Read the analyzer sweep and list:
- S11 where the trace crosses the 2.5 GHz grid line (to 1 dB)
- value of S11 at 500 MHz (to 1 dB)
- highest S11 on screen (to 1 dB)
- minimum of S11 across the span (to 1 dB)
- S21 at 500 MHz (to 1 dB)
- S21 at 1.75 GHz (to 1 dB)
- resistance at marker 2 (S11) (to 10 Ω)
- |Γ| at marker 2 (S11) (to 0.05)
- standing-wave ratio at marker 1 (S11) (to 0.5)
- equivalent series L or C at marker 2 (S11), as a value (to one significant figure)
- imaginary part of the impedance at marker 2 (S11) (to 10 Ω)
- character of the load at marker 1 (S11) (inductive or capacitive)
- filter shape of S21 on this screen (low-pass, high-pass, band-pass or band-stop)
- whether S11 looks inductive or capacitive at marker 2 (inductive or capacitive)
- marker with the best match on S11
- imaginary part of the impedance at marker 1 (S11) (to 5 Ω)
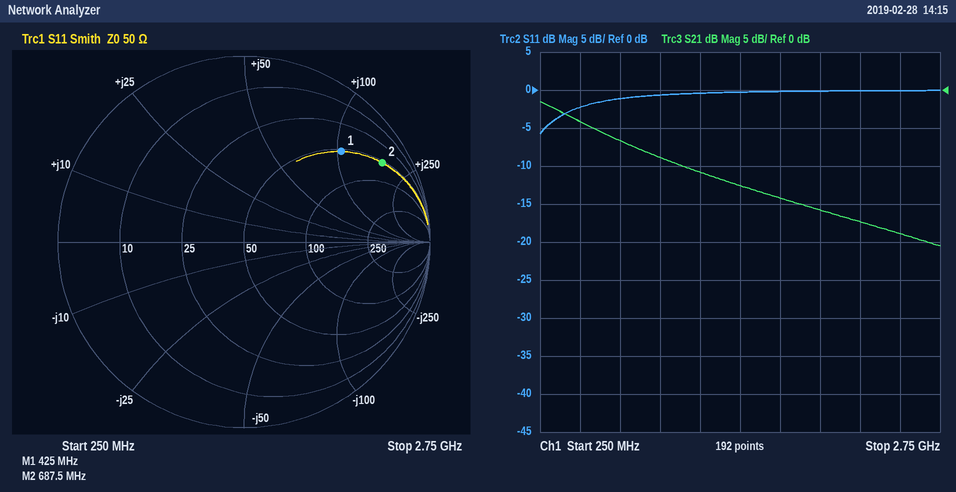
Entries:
0 dB
-2 dB
0 dB
-6 dB
-4 dB
-14 dB
50 Ω
0.85
6.0
40 nH
+170 Ω
inductive
low-pass
inductive
marker 1
+105 Ω
